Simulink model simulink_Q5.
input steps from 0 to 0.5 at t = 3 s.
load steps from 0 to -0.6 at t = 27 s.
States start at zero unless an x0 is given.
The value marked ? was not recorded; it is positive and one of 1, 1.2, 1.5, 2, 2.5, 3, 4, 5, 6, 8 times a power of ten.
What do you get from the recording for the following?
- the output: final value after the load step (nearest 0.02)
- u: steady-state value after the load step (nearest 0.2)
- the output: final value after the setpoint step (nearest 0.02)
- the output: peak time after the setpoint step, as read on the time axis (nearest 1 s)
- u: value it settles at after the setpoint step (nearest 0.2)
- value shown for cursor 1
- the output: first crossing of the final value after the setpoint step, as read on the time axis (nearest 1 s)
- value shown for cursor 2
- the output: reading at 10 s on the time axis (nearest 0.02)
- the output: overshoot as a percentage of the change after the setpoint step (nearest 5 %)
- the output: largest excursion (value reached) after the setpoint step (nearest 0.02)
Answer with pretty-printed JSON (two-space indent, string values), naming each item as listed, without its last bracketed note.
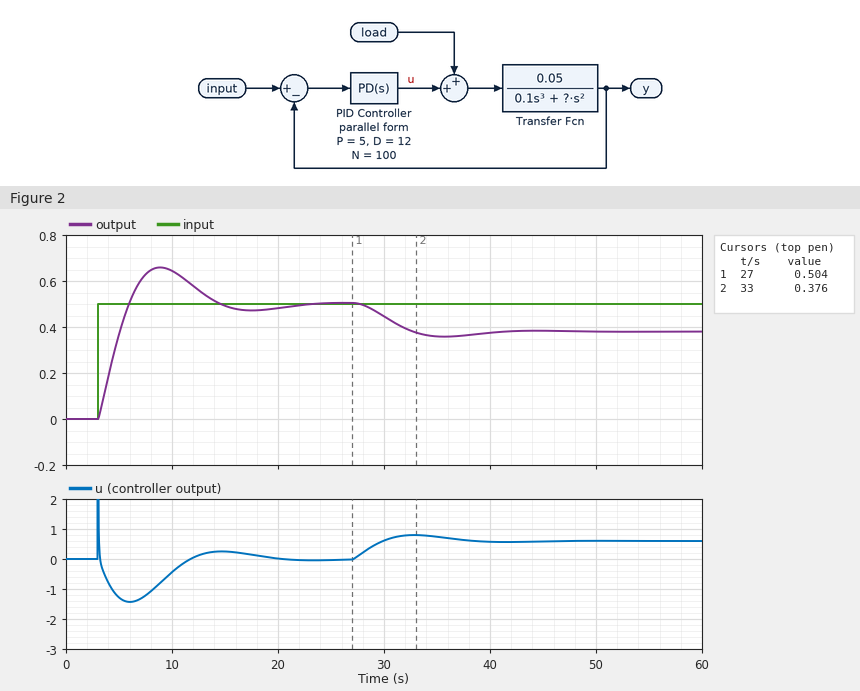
{
  "the output: final value after the load step": "0.38",
  "u: steady-state value after the load step": "0.6",
  "the output: final value after the setpoint step": "0.50",
  "the output: peak time after the setpoint step, as read on the time axis": "9 s",
  "u: value it settles at after the setpoint step": "0.0",
  "value shown for cursor 1": "0.504",
  "the output: first crossing of the final value after the setpoint step, as read on the time axis": "6 s",
  "value shown for cursor 2": "0.376",
  "the output: reading at 10 s on the time axis": "0.64",
  "the output: overshoot as a percentage of the change after the setpoint step": "30 %",
  "the output: largest excursion (value reached) after the setpoint step": "0.66"
}
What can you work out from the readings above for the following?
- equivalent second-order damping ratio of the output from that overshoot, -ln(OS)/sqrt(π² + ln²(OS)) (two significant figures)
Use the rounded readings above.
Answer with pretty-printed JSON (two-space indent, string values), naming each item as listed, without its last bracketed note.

{
  "equivalent second-order damping ratio of the output from that overshoot, -ln(OS)/sqrt(π² + ln²(OS))": "0.36"
}
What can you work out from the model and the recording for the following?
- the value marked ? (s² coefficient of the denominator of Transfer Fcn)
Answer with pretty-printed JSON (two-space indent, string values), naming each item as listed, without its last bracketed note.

{
  "the value marked ?": "1.5"
}
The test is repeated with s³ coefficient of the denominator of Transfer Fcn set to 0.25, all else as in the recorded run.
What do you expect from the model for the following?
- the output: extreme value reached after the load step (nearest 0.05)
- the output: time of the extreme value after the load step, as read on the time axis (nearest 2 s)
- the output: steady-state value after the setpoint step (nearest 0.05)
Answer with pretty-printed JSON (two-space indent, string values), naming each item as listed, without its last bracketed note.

{
  "the output: extreme value reached after the load step": "0.35",
  "the output: time of the extreme value after the load step, as read on the time axis": "36 s",
  "the output: steady-state value after the setpoint step": "0.50"
}
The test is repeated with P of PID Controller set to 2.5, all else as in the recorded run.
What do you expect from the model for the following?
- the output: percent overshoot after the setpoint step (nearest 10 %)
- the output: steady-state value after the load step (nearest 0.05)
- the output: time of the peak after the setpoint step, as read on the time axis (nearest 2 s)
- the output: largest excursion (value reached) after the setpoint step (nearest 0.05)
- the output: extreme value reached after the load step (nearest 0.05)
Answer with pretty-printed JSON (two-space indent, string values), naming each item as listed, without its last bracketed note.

{
  "the output: percent overshoot after the setpoint step": "20 %",
  "the output: steady-state value after the load step": "0.25",
  "the output: time of the peak after the setpoint step, as read on the time axis": "10 s",
  "the output: largest excursion (value reached) after the setpoint step": "0.60",
  "the output: extreme value reached after the load step": "0.25"
}
